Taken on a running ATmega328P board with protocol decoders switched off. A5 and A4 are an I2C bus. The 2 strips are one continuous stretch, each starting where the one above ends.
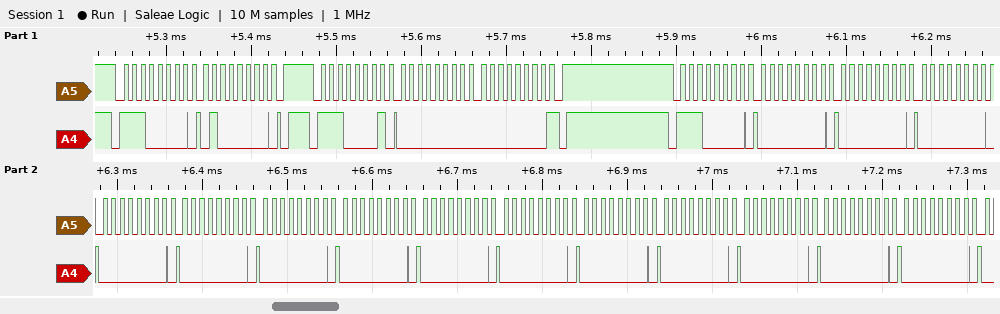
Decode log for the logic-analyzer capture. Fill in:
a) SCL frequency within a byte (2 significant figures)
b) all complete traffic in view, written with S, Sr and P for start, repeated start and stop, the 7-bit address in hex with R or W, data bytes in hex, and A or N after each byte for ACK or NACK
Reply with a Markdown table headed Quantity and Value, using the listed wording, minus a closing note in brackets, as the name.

| Quantity | Value |
|---|---|
| SCL frequency within a byte | 100 kHz |
| all complete traffic in view, written with S, Sr and P for start, repeated start and stop, the 7-bit address in hex with R or W, data bytes in hex, and A or N after each byte for ACK or NACK | S 70W A 40 A P S 70R A 00 A 00 N P S 70W A 00 A 00 A 00 A 00 A 00 A 00 A 00 A 00 A 00 A 00 A 00 A 00 A 00 A 00 A |
